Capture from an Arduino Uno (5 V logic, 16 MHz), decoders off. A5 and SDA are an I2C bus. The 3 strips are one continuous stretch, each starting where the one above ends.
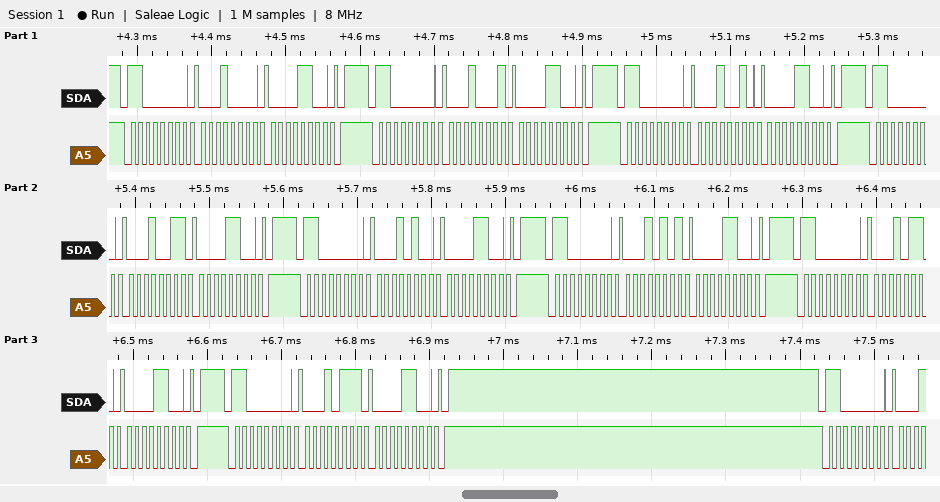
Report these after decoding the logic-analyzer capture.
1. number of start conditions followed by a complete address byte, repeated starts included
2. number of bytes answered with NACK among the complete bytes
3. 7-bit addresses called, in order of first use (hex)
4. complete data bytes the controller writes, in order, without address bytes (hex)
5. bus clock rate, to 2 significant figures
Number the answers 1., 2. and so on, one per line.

1. 9
2. 0
3. 0x60
4. 10 0C 11 0C 12 0C 13 0C 14 0C 15 0C 16 0C 17 0C
5. 100 kHz
